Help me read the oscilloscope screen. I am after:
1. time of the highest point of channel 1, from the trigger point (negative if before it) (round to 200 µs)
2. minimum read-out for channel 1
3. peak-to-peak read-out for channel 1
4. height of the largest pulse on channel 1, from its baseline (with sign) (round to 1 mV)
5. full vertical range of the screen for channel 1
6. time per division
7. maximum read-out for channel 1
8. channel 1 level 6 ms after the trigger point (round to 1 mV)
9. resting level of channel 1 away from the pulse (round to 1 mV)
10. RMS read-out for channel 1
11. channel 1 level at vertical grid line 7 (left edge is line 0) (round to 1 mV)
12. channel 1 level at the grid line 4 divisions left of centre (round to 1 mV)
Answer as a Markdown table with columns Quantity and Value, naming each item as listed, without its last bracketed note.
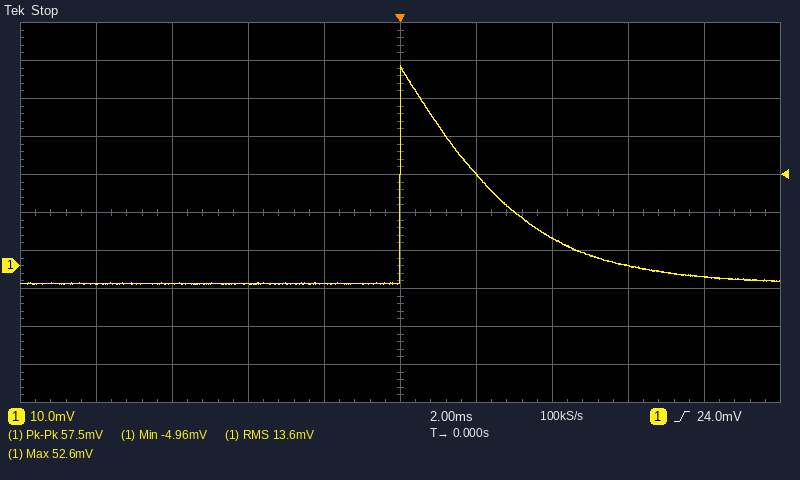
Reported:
| Quantity | Value |
|---|---|
| time of the highest point of channel 1, from the trigger point (negative if before it) | 0.0 ms |
| minimum read-out for channel 1 | -4.96 mV |
| peak-to-peak read-out for channel 1 | 57.5 mV |
| height of the largest pulse on channel 1, from its baseline (with sign) | +57 mV |
| full vertical range of the screen for channel 1 | 100 mV |
| time per division | 2 ms |
| maximum read-out for channel 1 | 52.6 mV |
| channel 1 level 6 ms after the trigger point | 0 mV |
| resting level of channel 1 away from the pulse | -5 mV |
| RMS read-out for channel 1 | 13.6 mV |
| channel 1 level at vertical grid line 7 (left edge is line 0) | 7 mV |
| channel 1 level at the grid line 4 divisions left of centre | -5 mV |
